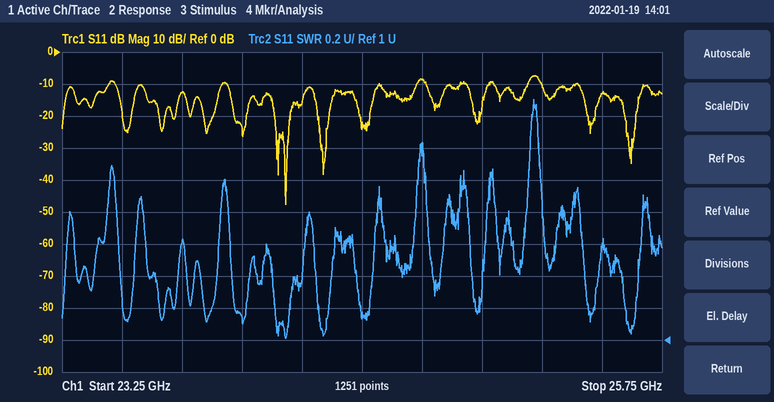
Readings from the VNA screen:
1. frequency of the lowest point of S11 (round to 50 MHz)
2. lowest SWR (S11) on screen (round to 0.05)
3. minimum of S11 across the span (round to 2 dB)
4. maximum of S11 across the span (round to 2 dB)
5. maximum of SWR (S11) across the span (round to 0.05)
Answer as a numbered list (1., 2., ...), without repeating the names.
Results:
1. 24.20 GHz
2. 1.00
3. -48 dB
4. -8 dB
5. 2.50
